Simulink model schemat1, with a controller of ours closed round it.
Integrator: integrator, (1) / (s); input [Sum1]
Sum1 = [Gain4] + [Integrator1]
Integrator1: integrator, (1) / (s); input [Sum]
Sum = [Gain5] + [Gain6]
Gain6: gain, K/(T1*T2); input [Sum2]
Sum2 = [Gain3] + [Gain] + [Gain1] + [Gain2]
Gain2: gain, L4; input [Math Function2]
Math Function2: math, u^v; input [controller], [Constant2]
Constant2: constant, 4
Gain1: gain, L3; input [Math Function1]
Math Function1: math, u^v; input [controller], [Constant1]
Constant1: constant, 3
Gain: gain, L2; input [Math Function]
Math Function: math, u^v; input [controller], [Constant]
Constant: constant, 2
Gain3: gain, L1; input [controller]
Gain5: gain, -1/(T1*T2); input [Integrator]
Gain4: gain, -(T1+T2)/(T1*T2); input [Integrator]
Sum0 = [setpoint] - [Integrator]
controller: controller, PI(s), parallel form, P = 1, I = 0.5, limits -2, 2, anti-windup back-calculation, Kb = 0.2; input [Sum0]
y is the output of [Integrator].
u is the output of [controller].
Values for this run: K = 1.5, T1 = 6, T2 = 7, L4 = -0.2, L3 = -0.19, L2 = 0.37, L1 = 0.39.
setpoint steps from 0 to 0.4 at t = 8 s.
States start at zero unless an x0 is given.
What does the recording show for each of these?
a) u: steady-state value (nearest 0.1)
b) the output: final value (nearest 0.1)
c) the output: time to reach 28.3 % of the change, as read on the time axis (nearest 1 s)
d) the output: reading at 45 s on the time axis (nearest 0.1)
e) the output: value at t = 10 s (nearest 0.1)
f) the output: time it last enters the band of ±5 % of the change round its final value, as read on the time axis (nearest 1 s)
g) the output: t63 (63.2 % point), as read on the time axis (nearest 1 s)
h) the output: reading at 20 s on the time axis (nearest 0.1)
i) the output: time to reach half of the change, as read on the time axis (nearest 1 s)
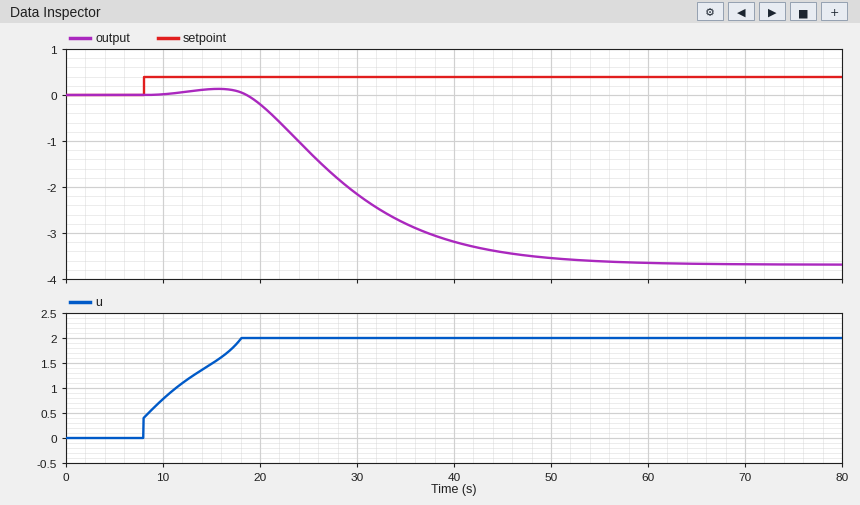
2.0
-3.7
24 s
-3.4
0.0
48 s
31 s
-0.2
28 s
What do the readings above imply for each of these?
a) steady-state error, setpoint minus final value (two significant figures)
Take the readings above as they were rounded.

4.1
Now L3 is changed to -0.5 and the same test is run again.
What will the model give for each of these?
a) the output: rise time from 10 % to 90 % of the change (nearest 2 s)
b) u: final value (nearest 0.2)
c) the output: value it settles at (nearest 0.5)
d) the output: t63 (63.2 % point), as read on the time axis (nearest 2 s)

22 s
2.0
-7.5
28 s
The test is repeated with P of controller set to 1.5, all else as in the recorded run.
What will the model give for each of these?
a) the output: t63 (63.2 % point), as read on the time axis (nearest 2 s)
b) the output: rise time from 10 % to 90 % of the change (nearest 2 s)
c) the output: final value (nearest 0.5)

30 s
22 s
-3.5
